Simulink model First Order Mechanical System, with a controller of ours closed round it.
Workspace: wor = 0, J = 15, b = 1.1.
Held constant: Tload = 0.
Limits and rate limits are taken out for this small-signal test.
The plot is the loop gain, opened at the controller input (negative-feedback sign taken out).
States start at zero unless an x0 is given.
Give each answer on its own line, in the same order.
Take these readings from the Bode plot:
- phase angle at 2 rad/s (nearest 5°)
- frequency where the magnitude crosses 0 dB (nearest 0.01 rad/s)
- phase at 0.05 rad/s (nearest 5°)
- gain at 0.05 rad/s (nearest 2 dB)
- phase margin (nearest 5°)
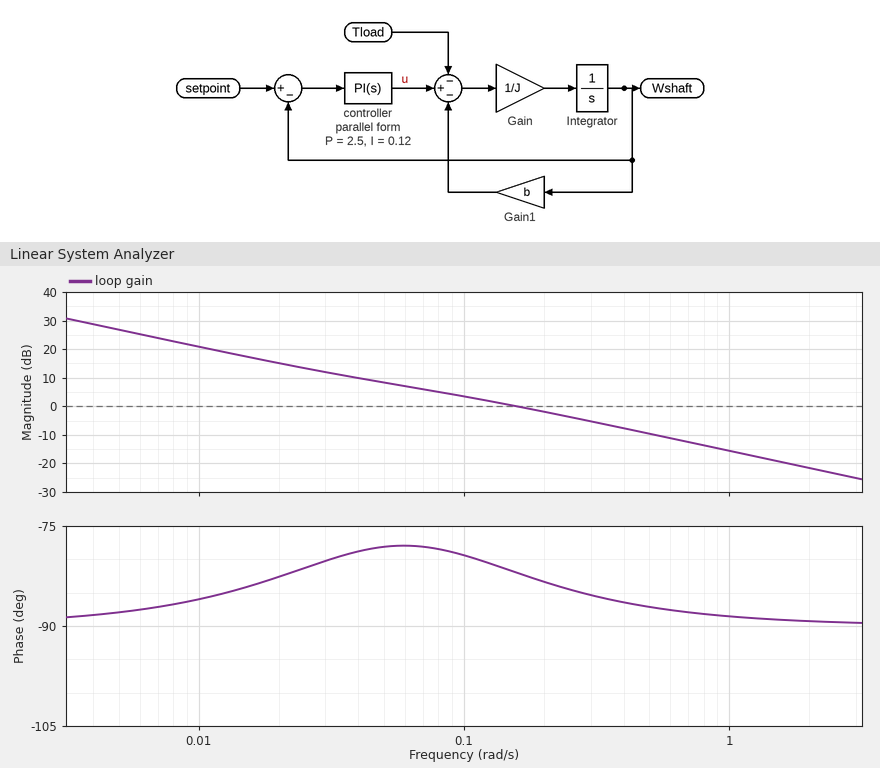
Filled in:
-90°
0.16 rad/s
-80°
8 dB
100°
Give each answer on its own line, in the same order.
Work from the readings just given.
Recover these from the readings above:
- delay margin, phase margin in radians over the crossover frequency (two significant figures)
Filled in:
11 s
